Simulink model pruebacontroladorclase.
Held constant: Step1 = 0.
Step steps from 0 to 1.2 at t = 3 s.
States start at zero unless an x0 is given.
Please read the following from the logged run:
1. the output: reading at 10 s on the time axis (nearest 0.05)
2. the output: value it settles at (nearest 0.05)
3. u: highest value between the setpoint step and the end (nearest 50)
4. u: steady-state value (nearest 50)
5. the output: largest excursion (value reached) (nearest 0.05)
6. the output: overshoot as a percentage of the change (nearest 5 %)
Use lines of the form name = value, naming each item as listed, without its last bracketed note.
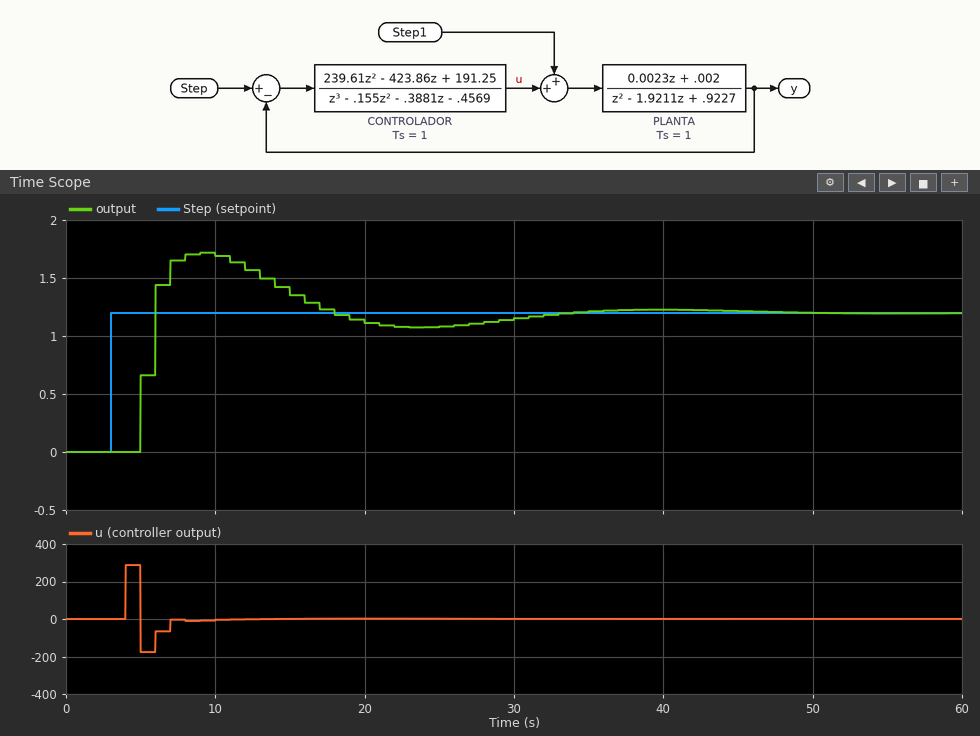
the output: reading at 10 s on the time axis = 1.70
the output: value it settles at = 1.20
u: highest value between the setpoint step and the end = 300
u: steady-state value = 0
the output: largest excursion (value reached) = 1.70
the output: overshoot as a percentage of the change = 45 %
